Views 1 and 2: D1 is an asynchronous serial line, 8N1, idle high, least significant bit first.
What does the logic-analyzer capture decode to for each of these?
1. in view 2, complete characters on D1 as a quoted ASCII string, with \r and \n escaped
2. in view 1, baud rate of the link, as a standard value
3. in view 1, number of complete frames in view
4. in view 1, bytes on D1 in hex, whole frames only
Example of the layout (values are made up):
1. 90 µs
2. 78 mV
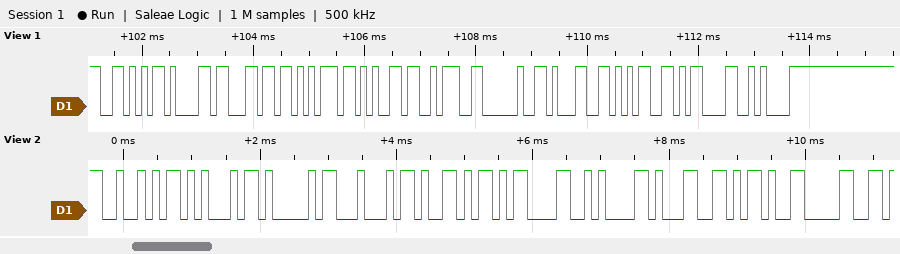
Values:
1. "READY\r\n1-0"
2. 9600 baud
3. 11
4. 56 61 6C 75 65 3A 20 31 35 0D 0A
